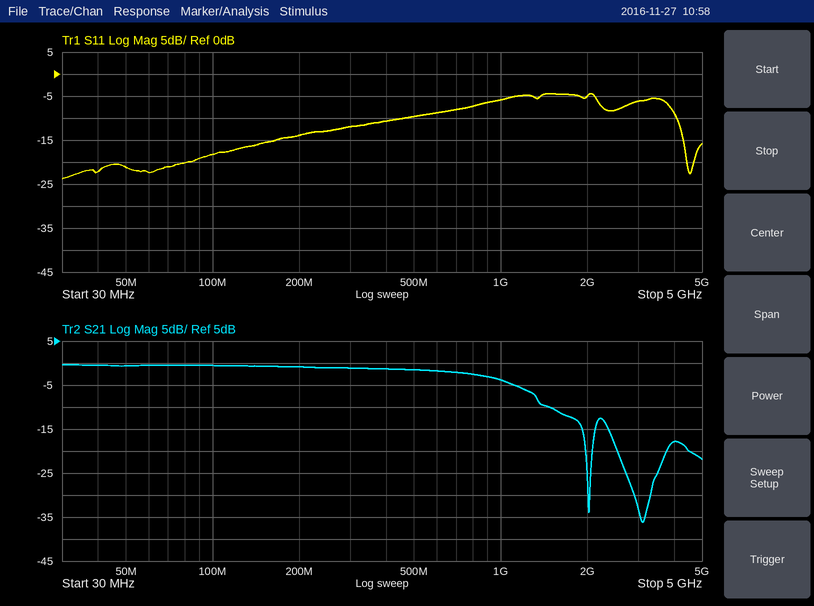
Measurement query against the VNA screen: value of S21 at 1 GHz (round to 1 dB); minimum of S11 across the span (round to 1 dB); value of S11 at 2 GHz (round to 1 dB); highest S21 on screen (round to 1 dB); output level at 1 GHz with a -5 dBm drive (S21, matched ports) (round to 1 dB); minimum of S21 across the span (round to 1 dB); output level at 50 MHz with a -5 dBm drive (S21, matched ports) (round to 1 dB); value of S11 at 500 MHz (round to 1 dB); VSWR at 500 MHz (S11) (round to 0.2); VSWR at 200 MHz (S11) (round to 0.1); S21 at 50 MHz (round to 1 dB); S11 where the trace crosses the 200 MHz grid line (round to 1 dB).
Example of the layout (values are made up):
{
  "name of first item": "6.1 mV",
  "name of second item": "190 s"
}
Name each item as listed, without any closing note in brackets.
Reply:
{
  "value of S21 at 1 GHz": "-4 dB",
  "minimum of S11 across the span": "-24 dB",
  "value of S11 at 2 GHz": "-5 dB",
  "highest S21 on screen": "0 dB",
  "output level at 1 GHz with a -5 dBm drive (S21, matched ports)": "-9 dBm",
  "minimum of S21 across the span": "-36 dB",
  "output level at 50 MHz with a -5 dBm drive (S21, matched ports)": "-6 dBm",
  "value of S11 at 500 MHz": "-10 dB",
  "VSWR at 500 MHz (S11)": "2.0",
  "VSWR at 200 MHz (S11)": "1.5",
  "S21 at 50 MHz": "-1 dB",
  "S11 where the trace crosses the 200 MHz grid line": "-14 dB"
}
